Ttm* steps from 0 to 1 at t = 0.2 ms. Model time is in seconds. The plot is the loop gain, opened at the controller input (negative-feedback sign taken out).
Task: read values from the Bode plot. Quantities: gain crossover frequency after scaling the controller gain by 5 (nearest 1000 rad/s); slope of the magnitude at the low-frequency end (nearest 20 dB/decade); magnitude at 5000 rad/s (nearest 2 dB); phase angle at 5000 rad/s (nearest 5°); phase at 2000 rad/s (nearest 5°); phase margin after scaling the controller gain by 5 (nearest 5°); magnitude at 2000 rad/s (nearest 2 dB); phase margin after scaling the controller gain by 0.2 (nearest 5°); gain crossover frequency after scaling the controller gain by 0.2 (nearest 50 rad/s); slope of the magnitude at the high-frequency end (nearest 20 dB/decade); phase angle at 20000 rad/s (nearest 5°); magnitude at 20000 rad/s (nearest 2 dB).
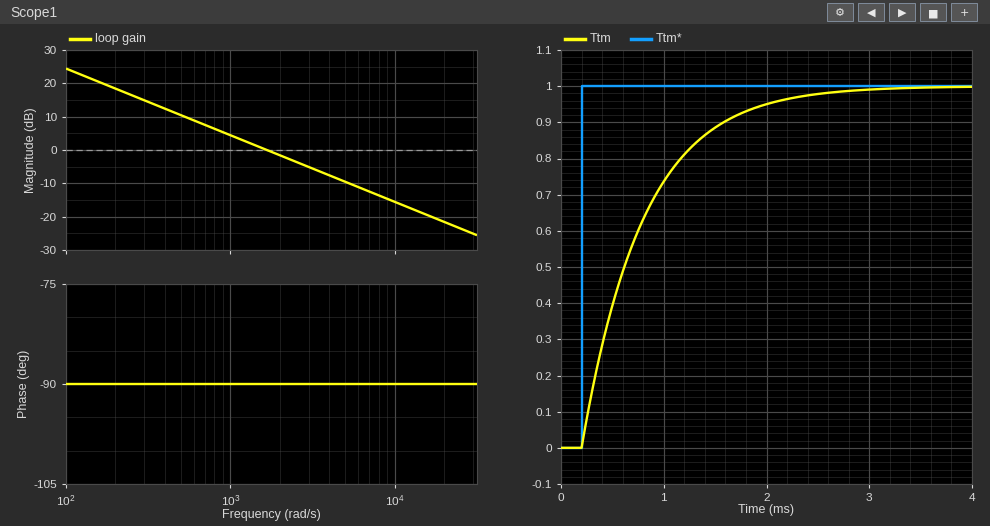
8000 rad/s
-20 dB/decade
-10 dB
-90°
-90°
90°
-2 dB
90°
350 rad/s
-20 dB/decade
-90°
-22 dB
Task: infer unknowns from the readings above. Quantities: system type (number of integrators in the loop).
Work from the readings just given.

1
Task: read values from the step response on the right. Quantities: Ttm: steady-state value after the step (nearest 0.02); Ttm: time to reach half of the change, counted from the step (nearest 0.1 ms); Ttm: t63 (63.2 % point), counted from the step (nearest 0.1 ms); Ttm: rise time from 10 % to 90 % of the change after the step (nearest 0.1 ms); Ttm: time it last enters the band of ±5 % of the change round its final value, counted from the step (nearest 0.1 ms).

1.00
0.4 ms
0.6 ms
1.3 ms
1.8 ms
